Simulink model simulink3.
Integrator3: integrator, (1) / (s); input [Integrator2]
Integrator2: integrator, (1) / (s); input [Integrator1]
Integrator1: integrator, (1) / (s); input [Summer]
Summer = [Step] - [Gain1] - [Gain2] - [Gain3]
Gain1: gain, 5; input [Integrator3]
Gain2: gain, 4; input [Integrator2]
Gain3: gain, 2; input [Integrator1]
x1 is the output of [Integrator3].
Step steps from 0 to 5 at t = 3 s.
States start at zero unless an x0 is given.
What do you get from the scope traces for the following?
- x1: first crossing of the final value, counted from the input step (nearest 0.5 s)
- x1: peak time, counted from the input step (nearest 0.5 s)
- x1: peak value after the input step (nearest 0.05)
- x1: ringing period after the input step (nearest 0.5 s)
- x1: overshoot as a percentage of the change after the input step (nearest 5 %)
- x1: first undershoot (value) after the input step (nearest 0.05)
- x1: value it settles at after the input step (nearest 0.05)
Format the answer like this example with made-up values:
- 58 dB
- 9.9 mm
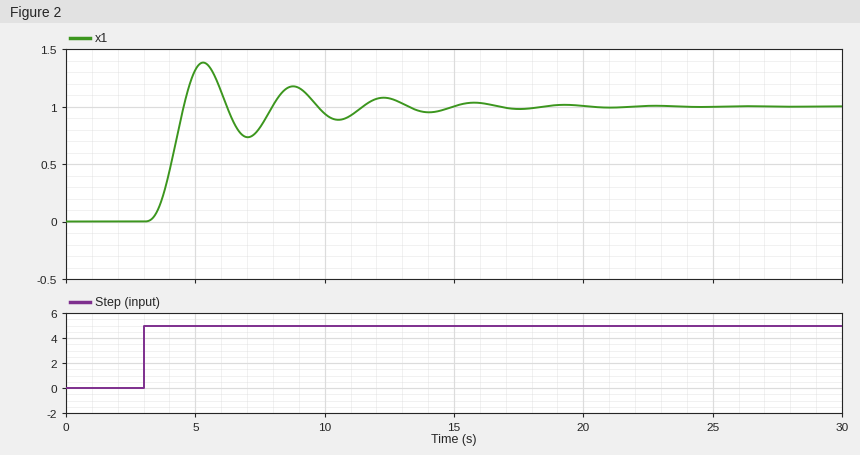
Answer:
- 1.5 s
- 2.5 s
- 1.40
- 3.5 s
- 40 %
- 0.75
- 1.00
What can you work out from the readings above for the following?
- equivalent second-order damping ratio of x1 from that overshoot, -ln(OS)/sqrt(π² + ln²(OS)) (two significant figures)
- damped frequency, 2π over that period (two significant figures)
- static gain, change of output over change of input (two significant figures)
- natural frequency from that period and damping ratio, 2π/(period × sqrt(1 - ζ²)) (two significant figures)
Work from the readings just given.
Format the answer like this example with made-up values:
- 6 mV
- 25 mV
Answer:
- 0.28
- 1.8 rad/s
- 0.20
- 1.9 rad/s
